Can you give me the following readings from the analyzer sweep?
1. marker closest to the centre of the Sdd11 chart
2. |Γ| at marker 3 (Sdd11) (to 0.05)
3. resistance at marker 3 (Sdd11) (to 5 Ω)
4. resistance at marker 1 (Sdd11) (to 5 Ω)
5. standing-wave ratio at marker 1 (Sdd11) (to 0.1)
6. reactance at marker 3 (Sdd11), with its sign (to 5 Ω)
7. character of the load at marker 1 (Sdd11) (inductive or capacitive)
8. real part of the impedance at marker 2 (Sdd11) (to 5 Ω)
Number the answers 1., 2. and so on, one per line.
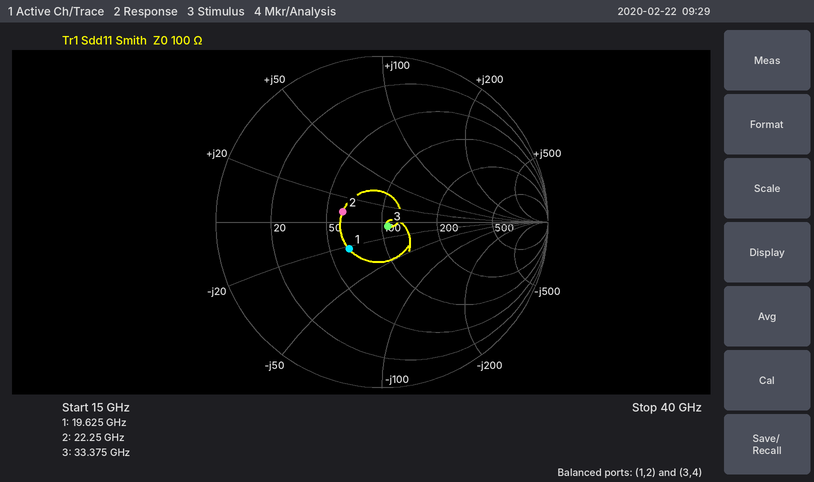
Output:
1. marker 3
2. 0.05
3. 105 Ω
4. 65 Ω
5. 1.7
6. -5 Ω
7. capacitive
8. 60 Ω
